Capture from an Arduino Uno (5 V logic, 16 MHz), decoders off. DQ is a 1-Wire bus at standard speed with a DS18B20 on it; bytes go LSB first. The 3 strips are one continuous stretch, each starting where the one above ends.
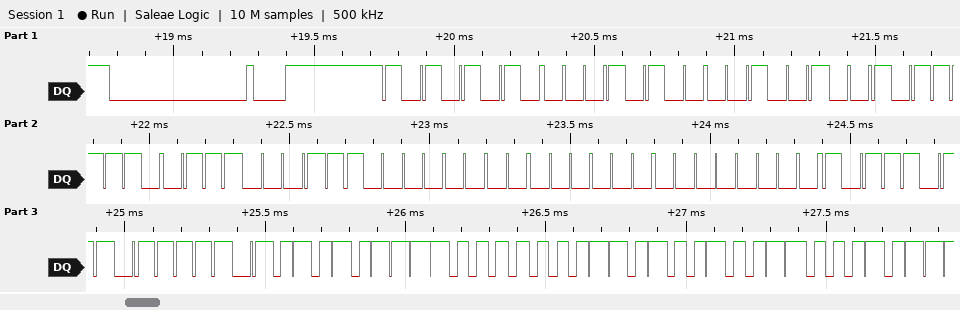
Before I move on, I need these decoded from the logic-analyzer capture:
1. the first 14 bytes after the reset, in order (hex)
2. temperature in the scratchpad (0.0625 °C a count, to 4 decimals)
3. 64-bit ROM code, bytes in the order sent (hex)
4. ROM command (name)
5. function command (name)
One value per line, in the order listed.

55 28 24 7D 8E 03 00 00 DD BE EA 01 4B 46
30.6250 °C
28 24 7D 8E 03 00 00 DD
Match ROM
Read Scratchpad
